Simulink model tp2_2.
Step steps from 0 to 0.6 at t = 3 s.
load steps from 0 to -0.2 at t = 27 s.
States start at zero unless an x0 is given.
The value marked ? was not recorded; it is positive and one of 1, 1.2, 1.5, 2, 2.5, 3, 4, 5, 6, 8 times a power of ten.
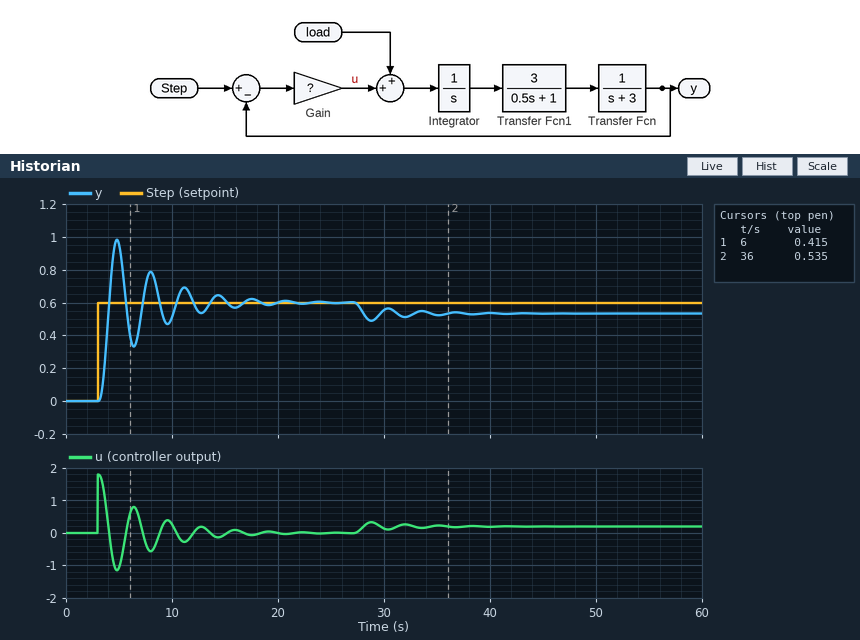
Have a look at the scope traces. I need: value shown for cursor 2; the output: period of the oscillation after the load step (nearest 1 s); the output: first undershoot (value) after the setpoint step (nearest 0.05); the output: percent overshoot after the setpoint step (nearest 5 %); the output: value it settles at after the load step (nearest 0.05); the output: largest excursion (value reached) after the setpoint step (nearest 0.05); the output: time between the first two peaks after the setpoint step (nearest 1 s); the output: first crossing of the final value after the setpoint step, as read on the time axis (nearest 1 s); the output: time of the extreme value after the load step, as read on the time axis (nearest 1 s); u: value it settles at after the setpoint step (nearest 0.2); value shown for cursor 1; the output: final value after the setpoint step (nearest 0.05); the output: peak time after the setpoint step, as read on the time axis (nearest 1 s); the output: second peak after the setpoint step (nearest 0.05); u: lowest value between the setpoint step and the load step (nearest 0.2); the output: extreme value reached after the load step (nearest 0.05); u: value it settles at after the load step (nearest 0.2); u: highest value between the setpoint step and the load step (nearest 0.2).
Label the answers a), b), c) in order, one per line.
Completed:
a) 0.535
b) 3 s
c) 0.35
d) 65 %
e) 0.55
f) 1.00
g) 3 s
h) 4 s
i) 29 s
j) 0.0
k) 0.415
l) 0.60
m) 5 s
n) 0.80
o) -1.2
p) 0.50
q) 0.2
r) 1.8
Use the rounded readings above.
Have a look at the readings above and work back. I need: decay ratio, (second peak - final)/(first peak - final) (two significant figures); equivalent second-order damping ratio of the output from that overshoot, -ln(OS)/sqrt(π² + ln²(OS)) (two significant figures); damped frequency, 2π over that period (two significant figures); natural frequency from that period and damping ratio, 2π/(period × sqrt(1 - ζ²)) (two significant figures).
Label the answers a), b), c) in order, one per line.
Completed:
a) 0.50
b) 0.14
c) 2.1 rad/s
d) 2.1 rad/s
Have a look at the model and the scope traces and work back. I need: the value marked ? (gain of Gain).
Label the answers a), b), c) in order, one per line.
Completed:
a) 3
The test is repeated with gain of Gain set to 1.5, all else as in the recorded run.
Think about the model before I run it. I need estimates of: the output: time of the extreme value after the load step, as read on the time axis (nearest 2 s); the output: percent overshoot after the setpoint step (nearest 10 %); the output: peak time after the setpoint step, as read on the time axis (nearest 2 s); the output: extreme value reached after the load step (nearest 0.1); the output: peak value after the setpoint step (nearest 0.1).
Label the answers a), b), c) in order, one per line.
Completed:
a) 30 s
b) 30 %
c) 6 s
d) 0.4
e) 0.8
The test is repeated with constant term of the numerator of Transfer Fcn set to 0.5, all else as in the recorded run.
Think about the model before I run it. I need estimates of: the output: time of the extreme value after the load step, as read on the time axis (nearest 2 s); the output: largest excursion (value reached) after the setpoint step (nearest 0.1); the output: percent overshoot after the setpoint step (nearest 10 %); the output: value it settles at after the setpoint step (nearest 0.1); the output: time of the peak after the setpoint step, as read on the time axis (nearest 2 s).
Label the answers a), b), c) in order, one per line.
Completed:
a) 30 s
b) 0.8
c) 30 %
d) 0.6
e) 6 s
